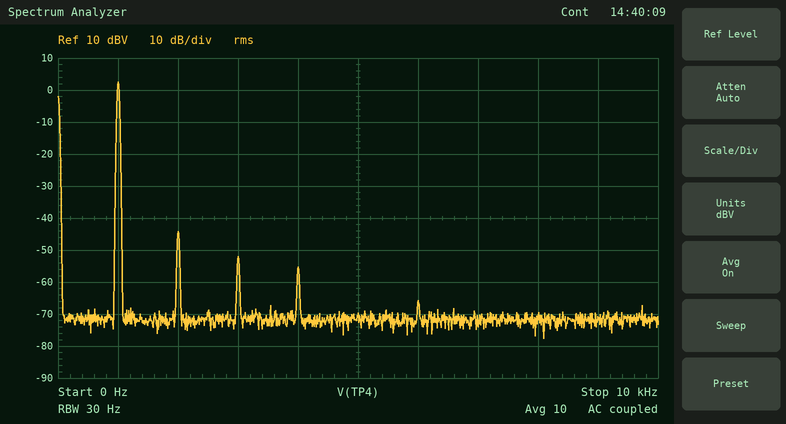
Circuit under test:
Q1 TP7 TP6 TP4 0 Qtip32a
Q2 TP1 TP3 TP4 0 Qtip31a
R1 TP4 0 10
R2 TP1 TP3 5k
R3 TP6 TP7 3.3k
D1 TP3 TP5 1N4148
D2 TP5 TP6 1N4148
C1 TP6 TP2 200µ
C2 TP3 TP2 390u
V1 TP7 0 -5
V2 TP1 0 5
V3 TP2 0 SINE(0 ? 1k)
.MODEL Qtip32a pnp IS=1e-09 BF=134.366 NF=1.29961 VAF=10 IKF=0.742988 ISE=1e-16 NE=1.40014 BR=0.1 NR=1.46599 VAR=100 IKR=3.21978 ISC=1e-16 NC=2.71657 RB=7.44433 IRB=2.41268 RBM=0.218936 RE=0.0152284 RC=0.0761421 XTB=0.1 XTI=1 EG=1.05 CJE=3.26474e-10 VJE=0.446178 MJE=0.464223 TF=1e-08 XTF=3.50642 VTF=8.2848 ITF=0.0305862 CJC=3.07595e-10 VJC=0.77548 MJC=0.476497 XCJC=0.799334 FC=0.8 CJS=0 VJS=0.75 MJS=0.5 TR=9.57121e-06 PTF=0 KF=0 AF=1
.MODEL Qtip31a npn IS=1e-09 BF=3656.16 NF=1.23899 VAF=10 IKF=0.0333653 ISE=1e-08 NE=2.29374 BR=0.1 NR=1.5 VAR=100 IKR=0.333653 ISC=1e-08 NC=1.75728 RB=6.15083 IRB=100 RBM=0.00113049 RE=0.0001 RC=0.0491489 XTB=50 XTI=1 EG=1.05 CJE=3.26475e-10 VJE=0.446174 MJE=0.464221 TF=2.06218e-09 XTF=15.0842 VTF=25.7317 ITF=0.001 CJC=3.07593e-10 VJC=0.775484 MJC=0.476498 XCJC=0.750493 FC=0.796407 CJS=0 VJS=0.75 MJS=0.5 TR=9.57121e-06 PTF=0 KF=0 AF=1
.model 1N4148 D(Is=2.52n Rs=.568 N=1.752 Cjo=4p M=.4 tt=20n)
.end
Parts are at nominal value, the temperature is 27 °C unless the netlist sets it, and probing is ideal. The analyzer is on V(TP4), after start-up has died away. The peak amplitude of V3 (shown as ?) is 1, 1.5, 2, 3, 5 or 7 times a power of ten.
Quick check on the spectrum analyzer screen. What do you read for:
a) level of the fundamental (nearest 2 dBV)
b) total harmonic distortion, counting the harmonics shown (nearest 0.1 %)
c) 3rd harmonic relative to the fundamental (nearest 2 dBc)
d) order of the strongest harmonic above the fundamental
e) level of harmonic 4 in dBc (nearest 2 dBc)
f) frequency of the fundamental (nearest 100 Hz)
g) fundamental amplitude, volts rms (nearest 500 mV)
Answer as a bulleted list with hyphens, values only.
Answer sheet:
- 2 dBV
- 0.5 %
- -54 dBc
- 2
- -58 dBc
- 1.0 kHz
- 1.5 V
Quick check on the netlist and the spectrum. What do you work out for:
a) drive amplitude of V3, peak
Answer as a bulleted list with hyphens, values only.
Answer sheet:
- 2 V
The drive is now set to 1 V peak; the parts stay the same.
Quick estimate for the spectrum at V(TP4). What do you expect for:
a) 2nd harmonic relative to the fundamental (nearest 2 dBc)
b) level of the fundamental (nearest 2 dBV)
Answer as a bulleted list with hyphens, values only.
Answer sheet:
- -48 dBc
- -4 dBV
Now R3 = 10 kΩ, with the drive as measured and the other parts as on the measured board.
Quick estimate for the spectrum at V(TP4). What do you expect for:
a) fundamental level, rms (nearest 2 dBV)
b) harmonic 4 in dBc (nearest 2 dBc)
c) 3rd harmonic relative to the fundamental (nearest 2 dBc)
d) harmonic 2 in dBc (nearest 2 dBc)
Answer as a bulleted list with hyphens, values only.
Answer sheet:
- 2 dBV
- -48 dBc
- -44 dBc
- -42 dBc
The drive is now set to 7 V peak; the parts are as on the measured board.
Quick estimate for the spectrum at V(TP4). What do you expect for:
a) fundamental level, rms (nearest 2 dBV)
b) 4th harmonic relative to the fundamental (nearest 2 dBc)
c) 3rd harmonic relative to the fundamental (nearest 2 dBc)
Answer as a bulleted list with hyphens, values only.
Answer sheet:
- 10 dBV
- -54 dBc
- -16 dBc
